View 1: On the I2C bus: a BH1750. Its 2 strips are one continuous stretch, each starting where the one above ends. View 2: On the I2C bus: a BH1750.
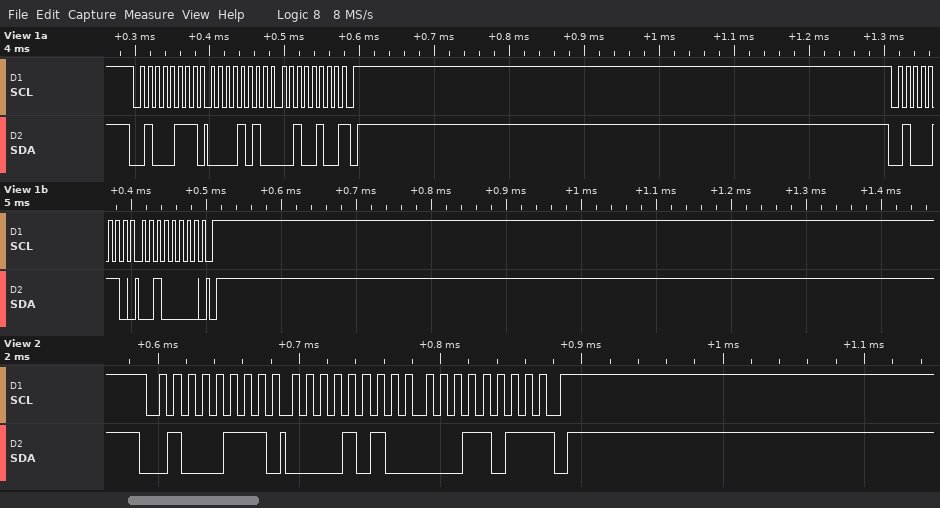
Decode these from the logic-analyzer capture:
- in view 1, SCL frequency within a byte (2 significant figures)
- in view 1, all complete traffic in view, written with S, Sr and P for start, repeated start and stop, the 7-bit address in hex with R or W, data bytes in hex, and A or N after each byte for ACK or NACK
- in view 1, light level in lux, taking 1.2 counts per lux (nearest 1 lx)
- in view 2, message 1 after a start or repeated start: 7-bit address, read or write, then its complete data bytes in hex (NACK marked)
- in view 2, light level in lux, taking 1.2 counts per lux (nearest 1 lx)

100 kHz
S 23R A 0A A 24 N P S 23W A 20 A P
2163 lx
0x23 read: 0A 1B NACK
2156 lx
